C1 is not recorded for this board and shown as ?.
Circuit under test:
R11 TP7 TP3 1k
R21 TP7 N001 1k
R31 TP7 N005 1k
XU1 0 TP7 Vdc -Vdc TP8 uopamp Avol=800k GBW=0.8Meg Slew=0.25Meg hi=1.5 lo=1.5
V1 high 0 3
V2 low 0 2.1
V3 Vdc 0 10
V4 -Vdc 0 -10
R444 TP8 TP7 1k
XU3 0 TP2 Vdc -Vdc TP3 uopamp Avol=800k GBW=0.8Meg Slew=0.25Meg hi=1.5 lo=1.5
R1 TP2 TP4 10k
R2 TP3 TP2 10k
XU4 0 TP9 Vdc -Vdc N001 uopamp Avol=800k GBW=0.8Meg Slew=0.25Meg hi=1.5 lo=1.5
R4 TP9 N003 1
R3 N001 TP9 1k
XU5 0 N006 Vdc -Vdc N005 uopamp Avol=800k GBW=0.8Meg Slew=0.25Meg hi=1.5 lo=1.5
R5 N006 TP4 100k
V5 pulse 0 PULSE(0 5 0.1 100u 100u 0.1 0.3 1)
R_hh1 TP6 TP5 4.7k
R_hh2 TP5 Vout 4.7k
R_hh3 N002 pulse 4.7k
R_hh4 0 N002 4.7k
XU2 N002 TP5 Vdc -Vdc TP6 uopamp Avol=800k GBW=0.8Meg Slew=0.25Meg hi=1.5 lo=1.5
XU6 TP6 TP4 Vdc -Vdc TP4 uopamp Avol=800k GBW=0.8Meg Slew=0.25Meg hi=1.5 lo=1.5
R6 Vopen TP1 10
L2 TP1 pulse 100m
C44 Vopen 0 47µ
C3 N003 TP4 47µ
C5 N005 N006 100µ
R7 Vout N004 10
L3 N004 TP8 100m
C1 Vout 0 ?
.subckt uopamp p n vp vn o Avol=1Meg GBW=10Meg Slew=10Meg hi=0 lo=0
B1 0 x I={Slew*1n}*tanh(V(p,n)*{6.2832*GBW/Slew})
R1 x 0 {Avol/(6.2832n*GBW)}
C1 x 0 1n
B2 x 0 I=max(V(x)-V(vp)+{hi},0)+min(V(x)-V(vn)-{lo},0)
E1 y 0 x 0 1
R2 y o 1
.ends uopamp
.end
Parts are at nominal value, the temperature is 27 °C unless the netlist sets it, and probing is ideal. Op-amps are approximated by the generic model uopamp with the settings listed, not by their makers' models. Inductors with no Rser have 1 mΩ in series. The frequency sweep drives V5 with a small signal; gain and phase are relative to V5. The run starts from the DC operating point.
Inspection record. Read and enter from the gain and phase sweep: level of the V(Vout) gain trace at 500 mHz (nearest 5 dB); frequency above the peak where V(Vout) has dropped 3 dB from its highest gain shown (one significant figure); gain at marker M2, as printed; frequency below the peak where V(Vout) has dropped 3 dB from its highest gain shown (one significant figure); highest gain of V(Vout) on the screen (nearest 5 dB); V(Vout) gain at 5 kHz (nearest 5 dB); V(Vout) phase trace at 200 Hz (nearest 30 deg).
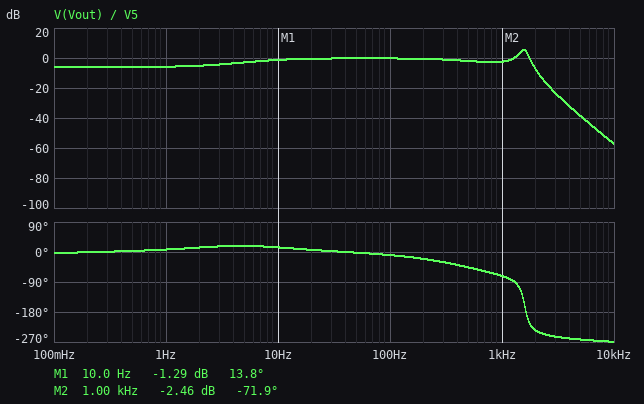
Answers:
-5 dB
2 kHz
-2.46 dB
1 kHz
5 dB
-40 dB
-30 deg
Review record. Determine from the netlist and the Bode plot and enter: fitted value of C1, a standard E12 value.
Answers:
150 µF
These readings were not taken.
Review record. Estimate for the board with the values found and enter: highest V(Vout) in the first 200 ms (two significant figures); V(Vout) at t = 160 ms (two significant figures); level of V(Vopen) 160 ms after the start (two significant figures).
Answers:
5.3 V
2.7 V
5.2 V
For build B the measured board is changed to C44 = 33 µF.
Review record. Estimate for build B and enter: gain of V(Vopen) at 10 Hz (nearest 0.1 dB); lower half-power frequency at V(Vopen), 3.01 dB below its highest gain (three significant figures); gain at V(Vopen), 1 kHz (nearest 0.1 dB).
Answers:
0.1 dB
78.5 Hz
-42.2 dB
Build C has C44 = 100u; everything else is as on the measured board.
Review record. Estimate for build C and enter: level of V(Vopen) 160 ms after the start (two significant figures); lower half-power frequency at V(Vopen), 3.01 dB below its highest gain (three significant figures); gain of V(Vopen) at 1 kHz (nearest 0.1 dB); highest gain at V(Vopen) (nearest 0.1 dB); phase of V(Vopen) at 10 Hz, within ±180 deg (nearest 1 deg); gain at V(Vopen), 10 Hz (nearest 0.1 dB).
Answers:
4.8 V
40.2 Hz
-51.9 dB
10.1 dB
-4 deg
0.3 dB
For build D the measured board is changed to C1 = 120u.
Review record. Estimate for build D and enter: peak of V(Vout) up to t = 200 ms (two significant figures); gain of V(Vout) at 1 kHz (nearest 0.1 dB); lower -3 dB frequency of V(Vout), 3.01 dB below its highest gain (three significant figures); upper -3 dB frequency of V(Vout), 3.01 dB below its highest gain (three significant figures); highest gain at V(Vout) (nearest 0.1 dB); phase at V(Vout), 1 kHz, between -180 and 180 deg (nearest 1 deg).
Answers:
5.5 V
-1.1 dB
1.52 kHz
1.68 kHz
12.0 dB
-62 deg
